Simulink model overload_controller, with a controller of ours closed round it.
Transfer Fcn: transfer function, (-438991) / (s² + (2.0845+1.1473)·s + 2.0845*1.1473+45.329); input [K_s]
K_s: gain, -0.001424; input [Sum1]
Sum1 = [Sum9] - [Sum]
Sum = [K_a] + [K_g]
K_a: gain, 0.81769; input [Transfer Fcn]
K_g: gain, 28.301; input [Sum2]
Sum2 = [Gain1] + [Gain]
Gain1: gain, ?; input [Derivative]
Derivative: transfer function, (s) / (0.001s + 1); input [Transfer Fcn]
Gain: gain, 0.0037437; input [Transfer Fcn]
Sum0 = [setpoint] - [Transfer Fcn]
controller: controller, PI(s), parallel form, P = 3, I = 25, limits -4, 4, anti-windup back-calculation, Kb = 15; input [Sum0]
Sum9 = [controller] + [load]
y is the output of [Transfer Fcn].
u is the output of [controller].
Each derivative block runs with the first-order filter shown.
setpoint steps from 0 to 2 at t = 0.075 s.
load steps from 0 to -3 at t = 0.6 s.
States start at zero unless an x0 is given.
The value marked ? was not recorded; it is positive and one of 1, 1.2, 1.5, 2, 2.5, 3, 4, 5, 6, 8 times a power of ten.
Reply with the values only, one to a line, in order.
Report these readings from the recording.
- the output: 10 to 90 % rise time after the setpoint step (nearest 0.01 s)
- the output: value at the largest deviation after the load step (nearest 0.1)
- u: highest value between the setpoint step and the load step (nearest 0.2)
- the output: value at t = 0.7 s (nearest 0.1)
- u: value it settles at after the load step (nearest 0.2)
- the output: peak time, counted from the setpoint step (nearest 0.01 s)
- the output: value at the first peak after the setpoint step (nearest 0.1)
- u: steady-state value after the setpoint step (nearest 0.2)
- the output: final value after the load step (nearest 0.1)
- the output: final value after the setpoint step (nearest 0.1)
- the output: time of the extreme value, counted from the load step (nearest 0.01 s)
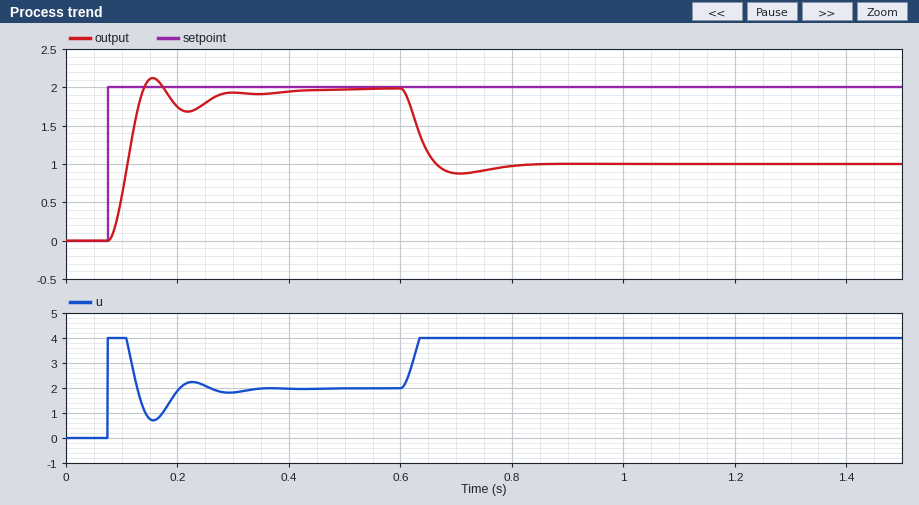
0.04 s
0.9
4.0
0.9
4.0
0.08 s
2.1
2.0
1.0
2.0
0.11 s
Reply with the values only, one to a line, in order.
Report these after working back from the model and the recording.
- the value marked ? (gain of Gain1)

0.002
